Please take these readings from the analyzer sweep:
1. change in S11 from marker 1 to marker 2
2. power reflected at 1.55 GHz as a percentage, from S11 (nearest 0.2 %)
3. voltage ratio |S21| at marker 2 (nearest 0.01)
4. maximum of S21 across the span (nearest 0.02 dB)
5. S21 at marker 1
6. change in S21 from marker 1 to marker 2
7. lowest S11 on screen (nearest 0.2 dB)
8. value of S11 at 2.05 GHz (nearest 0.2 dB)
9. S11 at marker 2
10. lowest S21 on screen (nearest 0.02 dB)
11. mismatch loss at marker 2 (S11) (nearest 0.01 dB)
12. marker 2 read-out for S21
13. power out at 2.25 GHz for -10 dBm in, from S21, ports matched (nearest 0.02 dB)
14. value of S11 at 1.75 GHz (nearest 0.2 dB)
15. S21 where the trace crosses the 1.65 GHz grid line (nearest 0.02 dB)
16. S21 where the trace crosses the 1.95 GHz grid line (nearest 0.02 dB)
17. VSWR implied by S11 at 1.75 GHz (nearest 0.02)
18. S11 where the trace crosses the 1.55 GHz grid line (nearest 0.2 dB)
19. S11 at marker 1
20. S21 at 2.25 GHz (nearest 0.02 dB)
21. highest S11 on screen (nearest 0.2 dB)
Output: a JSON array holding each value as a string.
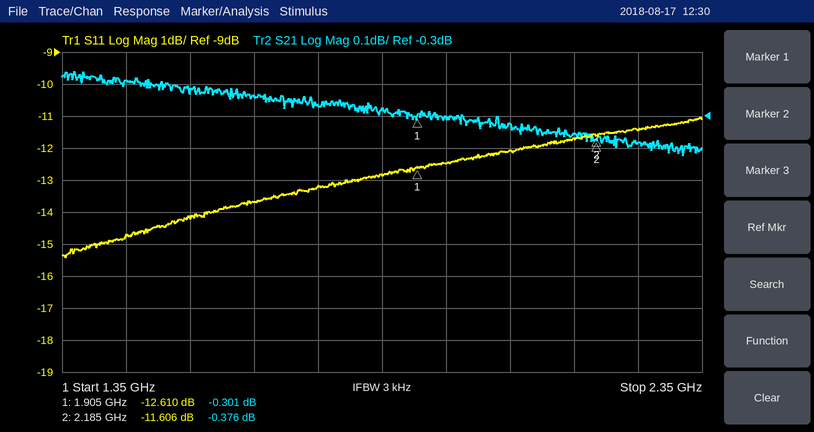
["1.004 dB", "3.8 %", "0.96", "-0.16 dB", "-0.301 dB", "-0.075 dB", "-15.4 dB", "-12.0 dB", "-11.606 dB", "-0.42 dB", "0.31 dB", "-0.376 dB", "-10.38 dBm", "-13.2 dB", "-0.24 dB", "-0.30 dB", "1.56", "-14.2 dB", "-12.610 dB", "-0.38 dB", "-11.0 dB"]
